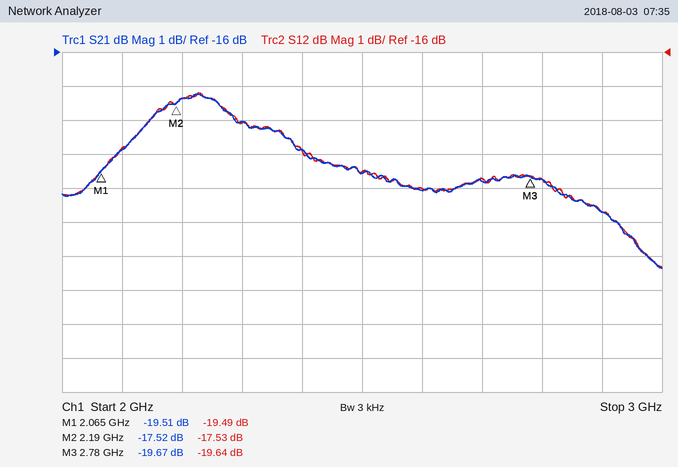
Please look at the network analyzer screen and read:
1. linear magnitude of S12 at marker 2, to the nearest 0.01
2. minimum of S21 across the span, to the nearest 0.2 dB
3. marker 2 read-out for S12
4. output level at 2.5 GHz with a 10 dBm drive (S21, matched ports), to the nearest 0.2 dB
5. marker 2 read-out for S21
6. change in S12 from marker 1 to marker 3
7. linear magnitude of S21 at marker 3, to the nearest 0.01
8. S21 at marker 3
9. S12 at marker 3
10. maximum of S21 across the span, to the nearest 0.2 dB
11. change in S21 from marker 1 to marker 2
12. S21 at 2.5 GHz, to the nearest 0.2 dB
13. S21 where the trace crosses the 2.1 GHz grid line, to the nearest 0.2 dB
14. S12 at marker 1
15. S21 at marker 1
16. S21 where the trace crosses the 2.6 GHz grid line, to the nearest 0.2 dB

0.13
-22.4 dB
-17.53 dB
-9.6 dBm
-17.52 dB
-0.15 dB
0.10
-19.67 dB
-19.64 dB
-17.2 dB
1.99 dB
-19.6 dB
-18.8 dB
-19.49 dB
-19.51 dB
-20.0 dB
